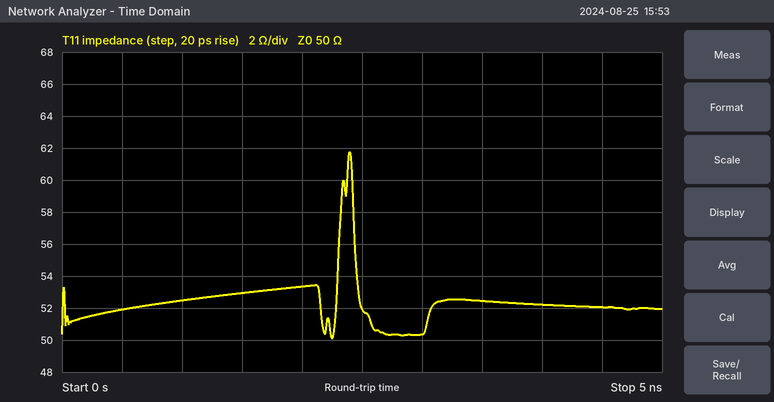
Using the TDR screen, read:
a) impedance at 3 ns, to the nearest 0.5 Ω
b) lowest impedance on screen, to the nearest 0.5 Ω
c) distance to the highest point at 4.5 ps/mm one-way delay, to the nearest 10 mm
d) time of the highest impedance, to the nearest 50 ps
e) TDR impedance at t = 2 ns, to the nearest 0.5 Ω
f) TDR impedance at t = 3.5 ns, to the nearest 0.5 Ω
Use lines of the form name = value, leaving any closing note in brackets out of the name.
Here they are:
impedance at 3 ns, to the nearest 0.5 Ω = 50.5 Ω
lowest impedance on screen, to the nearest 0.5 Ω = 50.0 Ω
distance to the highest point at 4.5 ps/mm one-way delay, to the nearest 10 mm = 270 mm
time of the highest impedance, to the nearest 50 ps = 2.40 ns
TDR impedance at t = 2 ns, to the nearest 0.5 Ω = 53.5 Ω
TDR impedance at t = 3.5 ns, to the nearest 0.5 Ω = 52.5 Ω
